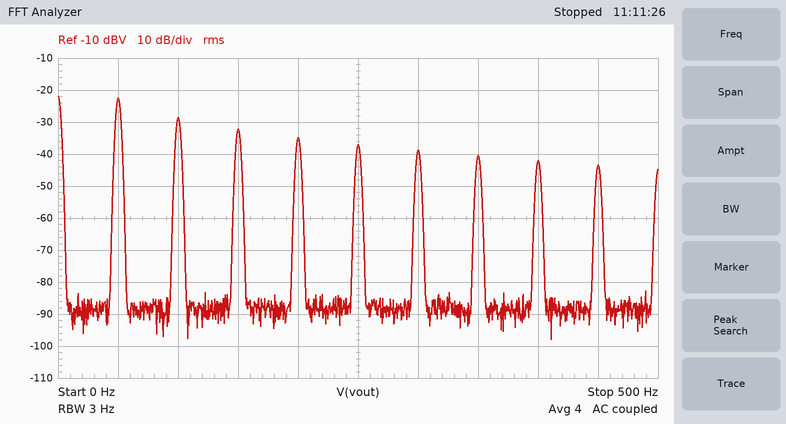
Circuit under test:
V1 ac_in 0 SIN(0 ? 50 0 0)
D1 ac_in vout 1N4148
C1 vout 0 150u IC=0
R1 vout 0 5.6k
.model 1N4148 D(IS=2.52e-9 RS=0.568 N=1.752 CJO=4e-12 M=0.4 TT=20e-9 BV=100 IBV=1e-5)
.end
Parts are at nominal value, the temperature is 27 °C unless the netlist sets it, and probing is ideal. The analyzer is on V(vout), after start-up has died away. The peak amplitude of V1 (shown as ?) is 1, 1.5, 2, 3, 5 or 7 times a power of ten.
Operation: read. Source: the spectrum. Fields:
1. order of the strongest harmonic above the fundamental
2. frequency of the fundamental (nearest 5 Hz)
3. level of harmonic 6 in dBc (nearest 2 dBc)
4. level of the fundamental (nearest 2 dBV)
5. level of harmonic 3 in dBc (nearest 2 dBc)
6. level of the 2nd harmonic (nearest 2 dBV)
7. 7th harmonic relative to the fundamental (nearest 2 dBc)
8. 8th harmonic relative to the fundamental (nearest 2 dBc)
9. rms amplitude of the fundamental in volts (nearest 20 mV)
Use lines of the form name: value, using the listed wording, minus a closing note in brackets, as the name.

order of the strongest harmonic above the fundamental: 2
frequency of the fundamental: 50 Hz
level of harmonic 6 in dBc: -16 dBc
level of the fundamental: -22 dBV
level of harmonic 3 in dBc: -10 dBc
level of the 2nd harmonic: -28 dBV
7th harmonic relative to the fundamental: -18 dBc
8th harmonic relative to the fundamental: -20 dBc
rms amplitude of the fundamental in volts: 80 mV
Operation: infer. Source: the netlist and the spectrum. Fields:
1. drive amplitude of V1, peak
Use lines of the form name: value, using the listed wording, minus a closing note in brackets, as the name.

drive amplitude of V1, peak: 15 V
